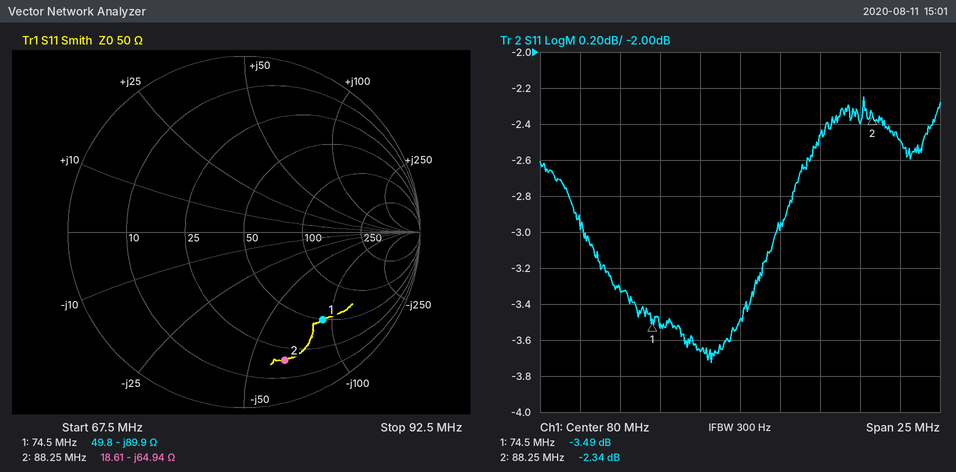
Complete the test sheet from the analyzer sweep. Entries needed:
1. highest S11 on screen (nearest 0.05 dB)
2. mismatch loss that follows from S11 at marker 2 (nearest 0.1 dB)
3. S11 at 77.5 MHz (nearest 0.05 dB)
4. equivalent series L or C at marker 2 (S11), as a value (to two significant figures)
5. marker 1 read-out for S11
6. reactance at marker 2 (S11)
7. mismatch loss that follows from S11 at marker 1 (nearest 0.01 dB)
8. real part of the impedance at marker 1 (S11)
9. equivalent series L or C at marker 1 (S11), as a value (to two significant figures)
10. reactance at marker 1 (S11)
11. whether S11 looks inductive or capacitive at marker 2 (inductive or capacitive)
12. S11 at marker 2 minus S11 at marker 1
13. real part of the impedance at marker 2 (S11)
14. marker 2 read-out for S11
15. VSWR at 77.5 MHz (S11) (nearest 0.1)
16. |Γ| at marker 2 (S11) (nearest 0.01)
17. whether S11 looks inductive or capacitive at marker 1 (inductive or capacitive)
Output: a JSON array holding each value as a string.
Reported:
["-2.25 dB", "3.8 dB", "-3.65 dB", "28 pF", "-3.49 dB", "-64.94 Ω", "2.58 dB", "49.8 Ω", "24 pF", "-89.9 Ω", "capacitive", "1.15 dB", "18.61 Ω", "-2.34 dB", "4.8", "0.76", "capacitive"]
